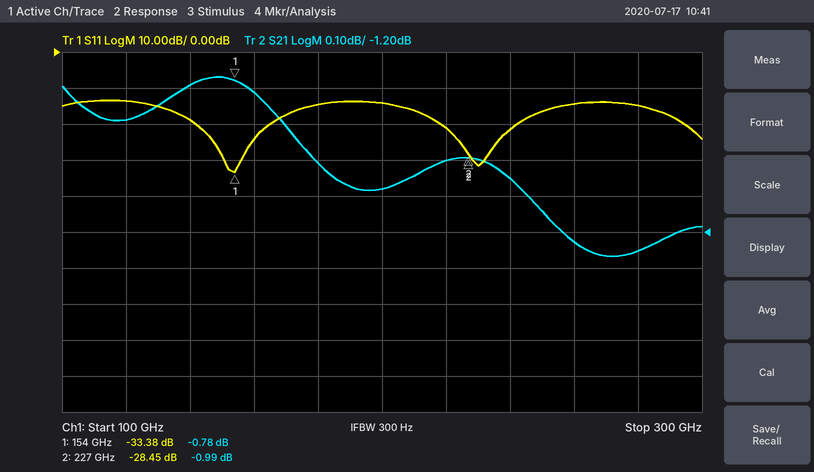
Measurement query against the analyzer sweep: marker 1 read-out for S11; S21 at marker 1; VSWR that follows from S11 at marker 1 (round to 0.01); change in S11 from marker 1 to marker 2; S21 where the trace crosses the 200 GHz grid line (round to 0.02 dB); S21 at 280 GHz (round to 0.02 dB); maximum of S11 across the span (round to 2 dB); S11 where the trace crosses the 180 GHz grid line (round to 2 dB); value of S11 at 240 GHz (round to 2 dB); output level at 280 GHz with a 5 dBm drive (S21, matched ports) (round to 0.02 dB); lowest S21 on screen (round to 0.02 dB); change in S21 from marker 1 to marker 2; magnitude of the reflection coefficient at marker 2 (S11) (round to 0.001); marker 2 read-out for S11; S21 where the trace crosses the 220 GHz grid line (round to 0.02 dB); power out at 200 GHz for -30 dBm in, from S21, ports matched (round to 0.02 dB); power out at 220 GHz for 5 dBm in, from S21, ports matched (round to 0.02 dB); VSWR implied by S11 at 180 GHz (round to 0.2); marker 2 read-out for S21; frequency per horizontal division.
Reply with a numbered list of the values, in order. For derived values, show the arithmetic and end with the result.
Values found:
1. -33.38 dB
2. -0.78 dB
3. (1 + 0.0214)/(1 − 0.0214) ≈ 1.04
4. -28.45 − (-33.38) = 4.93 dB
5. -1.08 dB
6. -1.26 dB
7. -14 dB
8. -14 dB
9. -22 dB
10. 5 dBm + (-1.26 dB) = 3.74 dBm
11. -1.26 dB
12. -0.99 − (-0.78) = -0.21 dB
13. 10^(-28.45/20) ≈ 0.038
14. -28.45 dB
15. -1.00 dB
16. -30 dBm + (-1.08 dB) = -31.08 dBm
17. 5 dBm + (-1.00 dB) = 4.00 dBm
18. |Γ| = 10^(-14/20) = 0.1995; VSWR = (1 + 0.1995)/(1 − 0.1995) ≈ 1.50, so 1.4 to the nearest 0.2
19. -0.99 dB
20. 20 GHz
